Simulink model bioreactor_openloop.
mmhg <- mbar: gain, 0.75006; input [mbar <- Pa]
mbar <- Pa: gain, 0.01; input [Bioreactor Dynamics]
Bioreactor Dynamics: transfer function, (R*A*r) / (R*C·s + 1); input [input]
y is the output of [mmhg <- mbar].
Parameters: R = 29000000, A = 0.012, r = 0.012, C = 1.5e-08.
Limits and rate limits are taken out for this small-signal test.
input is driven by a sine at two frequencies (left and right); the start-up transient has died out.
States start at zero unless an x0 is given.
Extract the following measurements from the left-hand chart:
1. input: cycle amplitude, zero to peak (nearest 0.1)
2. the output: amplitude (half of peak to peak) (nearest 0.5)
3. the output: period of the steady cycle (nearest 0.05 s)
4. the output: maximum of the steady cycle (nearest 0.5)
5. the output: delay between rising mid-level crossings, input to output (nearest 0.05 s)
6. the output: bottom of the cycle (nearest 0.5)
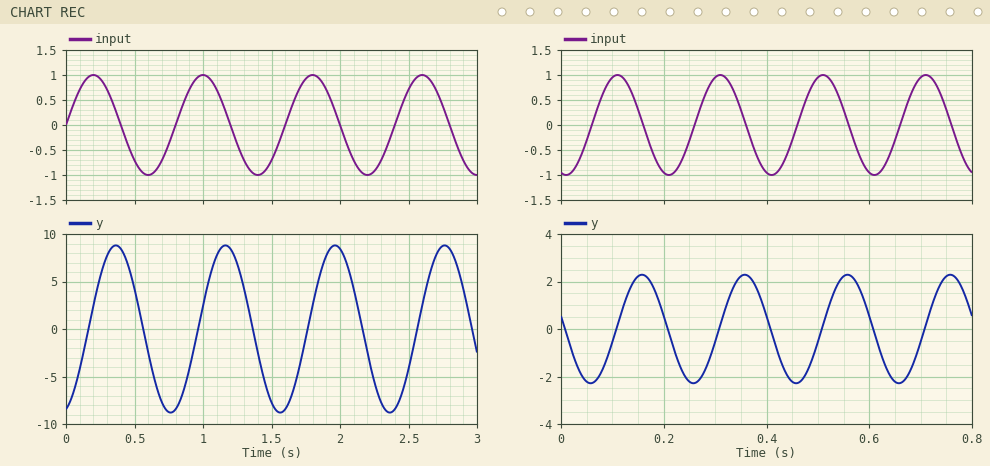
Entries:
1.0
9.0
0.80 s
9.0
0.15 s
-9.0
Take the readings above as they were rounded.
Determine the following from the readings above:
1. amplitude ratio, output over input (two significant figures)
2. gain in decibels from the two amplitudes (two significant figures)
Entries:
9.0
19 dB
